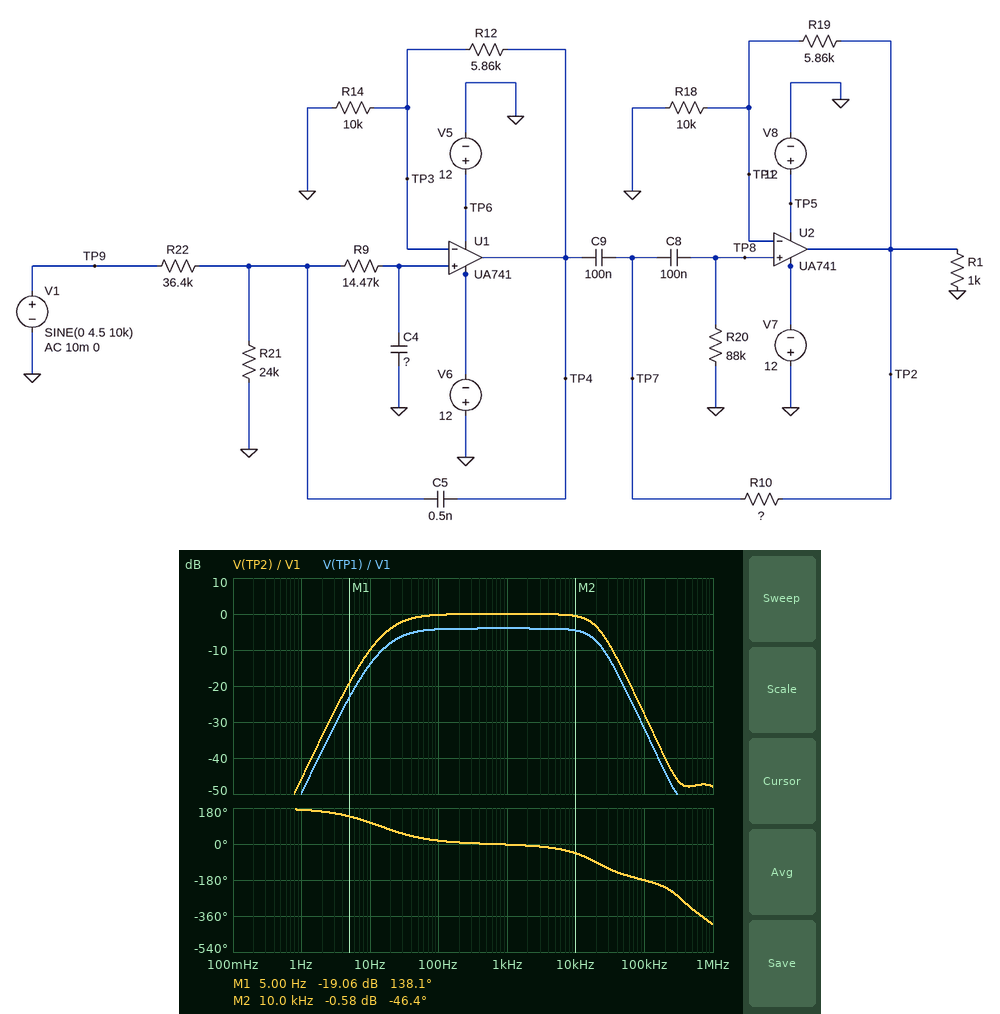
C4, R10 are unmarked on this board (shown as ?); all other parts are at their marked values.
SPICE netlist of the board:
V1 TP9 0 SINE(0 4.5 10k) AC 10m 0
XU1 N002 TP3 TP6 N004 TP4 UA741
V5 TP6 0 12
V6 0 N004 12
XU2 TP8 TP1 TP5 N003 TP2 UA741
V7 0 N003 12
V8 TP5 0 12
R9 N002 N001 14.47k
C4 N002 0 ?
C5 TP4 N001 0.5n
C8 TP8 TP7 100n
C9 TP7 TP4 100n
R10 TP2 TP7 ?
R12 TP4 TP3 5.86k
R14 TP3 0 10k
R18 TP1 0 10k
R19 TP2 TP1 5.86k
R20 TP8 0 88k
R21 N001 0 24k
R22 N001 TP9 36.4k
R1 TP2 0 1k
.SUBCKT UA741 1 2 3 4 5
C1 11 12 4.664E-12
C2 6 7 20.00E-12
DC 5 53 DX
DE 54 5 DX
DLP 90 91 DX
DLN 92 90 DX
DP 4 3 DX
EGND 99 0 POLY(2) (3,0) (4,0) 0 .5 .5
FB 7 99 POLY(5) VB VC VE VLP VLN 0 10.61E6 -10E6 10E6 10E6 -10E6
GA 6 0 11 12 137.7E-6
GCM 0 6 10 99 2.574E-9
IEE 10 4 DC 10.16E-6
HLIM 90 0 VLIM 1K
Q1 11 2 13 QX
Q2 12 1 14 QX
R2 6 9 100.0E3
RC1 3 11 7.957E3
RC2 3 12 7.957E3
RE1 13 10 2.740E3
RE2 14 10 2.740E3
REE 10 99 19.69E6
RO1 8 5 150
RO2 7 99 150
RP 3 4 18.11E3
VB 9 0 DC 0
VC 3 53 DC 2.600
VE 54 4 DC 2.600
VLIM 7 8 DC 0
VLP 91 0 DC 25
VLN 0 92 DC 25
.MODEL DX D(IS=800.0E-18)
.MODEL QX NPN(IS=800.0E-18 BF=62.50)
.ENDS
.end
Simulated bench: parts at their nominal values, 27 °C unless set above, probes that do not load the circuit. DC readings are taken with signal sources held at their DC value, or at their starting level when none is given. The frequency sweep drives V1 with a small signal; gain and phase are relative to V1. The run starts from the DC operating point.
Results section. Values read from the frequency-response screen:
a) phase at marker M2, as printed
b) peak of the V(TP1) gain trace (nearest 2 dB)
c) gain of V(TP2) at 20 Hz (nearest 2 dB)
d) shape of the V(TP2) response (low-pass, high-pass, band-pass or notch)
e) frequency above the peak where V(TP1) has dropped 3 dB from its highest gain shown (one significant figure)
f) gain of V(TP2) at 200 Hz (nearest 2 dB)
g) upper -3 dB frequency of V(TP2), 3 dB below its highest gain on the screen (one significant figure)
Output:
-46.4 deg
-4 dB
-4 dB
band-pass
20 kHz
0 dB
20 kHz
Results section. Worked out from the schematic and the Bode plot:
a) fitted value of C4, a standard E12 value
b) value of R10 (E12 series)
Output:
560 pF
150 kΩ
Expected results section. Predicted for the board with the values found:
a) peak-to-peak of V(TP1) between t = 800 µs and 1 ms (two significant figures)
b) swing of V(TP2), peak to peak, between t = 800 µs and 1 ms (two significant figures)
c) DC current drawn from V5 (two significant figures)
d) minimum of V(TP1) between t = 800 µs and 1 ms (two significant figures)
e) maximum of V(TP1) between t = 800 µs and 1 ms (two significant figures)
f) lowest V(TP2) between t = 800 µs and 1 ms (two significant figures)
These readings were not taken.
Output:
5.3 V
8.4 V
1.3 mA
-2.7 V
2.6 V
-4.2 V
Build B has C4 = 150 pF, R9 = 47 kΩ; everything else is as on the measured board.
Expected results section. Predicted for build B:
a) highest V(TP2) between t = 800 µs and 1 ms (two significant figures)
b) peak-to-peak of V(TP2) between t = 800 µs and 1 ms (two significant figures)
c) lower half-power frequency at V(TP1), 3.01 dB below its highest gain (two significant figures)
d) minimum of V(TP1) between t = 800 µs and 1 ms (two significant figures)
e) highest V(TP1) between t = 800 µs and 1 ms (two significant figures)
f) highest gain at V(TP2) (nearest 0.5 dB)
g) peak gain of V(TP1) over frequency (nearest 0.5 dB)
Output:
5.3 V
11 V
7.7 kHz
-3.4 V
3.3 V
4.0 dB
0 dB
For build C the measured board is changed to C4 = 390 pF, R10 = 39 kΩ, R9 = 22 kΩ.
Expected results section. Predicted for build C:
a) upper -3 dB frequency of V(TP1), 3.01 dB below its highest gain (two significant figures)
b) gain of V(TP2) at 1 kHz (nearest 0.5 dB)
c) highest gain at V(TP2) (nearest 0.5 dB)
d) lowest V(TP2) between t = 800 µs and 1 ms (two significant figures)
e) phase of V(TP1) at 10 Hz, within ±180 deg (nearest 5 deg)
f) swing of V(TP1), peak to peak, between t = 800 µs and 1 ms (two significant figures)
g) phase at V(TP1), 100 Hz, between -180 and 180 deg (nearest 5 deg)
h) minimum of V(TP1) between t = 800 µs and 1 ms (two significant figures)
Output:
40 Hz
0 dB
7.0 dB
-4.6 V
170 deg
5.8 V
5 deg
-2.9 V
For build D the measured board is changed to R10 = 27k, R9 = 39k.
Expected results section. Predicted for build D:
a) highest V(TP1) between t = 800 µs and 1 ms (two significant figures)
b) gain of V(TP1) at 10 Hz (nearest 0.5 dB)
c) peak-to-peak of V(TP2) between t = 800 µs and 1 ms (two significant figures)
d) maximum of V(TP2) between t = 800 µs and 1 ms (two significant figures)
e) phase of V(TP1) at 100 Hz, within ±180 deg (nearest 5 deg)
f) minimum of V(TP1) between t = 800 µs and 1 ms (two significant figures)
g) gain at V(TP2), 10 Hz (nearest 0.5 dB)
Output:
1.7 V
-23.5 dB
5.4 V
2.7 V
0 deg
-1.7 V
-19.5 dB
